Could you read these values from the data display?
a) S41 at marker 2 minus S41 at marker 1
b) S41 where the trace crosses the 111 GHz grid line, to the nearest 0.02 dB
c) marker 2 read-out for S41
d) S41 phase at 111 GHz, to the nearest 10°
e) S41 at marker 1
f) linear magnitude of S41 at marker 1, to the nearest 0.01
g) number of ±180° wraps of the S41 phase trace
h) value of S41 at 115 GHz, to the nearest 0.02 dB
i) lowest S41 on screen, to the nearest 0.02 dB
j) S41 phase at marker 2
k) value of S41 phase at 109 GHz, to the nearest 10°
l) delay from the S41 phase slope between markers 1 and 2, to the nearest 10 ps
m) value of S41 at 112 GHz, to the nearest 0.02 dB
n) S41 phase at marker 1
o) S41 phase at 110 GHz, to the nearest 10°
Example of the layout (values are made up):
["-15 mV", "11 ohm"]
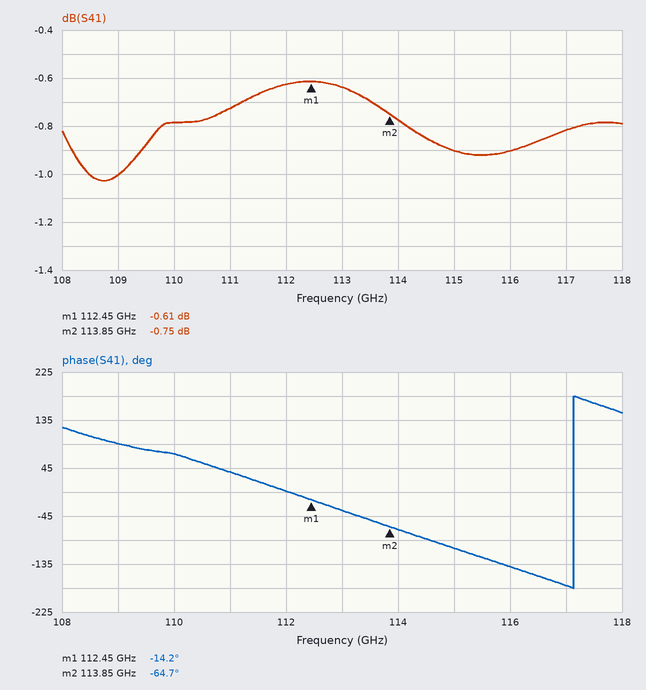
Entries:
["-0.14 dB", "-0.72 dB", "-0.75 dB", "40°", "-0.61 dB", "0.93", "1", "-0.90 dB", "-1.02 dB", "-64.7°", "90°", "100 ps", "-0.62 dB", "-14.2°", "70°"]
